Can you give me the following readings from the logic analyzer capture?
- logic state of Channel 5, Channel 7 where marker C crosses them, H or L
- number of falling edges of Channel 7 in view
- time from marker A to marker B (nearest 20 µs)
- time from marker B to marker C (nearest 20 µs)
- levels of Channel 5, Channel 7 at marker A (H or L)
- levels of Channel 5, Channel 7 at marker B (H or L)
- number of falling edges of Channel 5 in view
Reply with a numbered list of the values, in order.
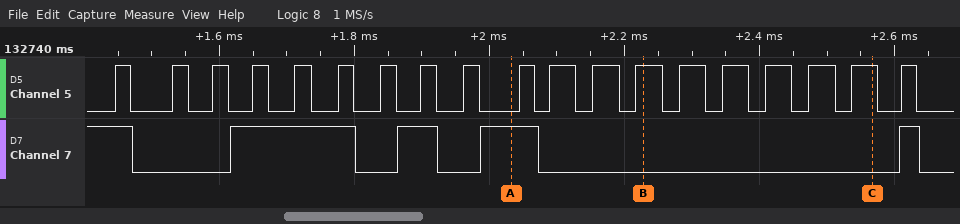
1. Channel 5=H, Channel 7=L
2. 5
3. 200 µs
4. 340 µs
5. Channel 5=L, Channel 7=H
6. Channel 5=H, Channel 7=L
7. 19
